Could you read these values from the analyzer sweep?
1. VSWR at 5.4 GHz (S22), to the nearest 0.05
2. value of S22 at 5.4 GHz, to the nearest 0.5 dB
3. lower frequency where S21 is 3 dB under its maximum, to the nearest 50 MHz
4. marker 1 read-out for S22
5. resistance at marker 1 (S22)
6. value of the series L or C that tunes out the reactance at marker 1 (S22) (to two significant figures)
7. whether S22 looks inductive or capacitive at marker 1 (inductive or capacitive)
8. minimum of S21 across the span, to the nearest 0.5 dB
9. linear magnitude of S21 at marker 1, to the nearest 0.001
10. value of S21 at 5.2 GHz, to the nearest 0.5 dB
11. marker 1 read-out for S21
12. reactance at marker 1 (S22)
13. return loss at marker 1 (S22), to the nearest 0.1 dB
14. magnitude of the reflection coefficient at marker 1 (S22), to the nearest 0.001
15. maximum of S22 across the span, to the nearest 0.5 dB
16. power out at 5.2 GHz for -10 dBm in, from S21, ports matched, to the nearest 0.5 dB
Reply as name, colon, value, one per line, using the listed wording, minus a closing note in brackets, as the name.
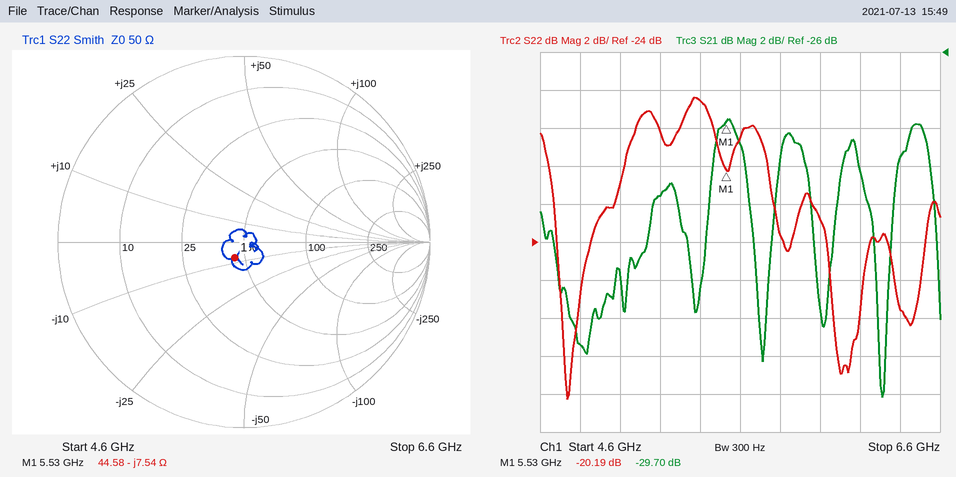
VSWR at 5.4 GHz (S22), to the nearest 0.05: 1.35
value of S22 at 5.4 GHz, to the nearest 0.5 dB: -16.5 dB
lower frequency where S21 is 3 dB under its maximum, to the nearest 50 MHz: 5.45 GHz
marker 1 read-out for S22: -20.19 dB
resistance at marker 1: 44.58 Ω
value of the series L or C that tunes out the reactance at marker 1 (S22): 220 pH
whether S22 looks inductive or capacitive at marker 1: capacitive
minimum of S21 across the span, to the nearest 0.5 dB: -44.0 dB
linear magnitude of S21 at marker 1, to the nearest 0.001: 0.033
value of S21 at 5.2 GHz, to the nearest 0.5 dB: -33.5 dB
marker 1 read-out for S21: -29.70 dB
reactance at marker 1: -7.54 Ω
return loss at marker 1 (S22), to the nearest 0.1 dB: 20.2 dB
magnitude of the reflection coefficient at marker 1 (S22), to the nearest 0.001: 0.098
maximum of S22 across the span, to the nearest 0.5 dB: -16.5 dB
power out at 5.2 GHz for -10 dBm in, from S21, ports matched, to the nearest 0.5 dB: -43.5 dBm
